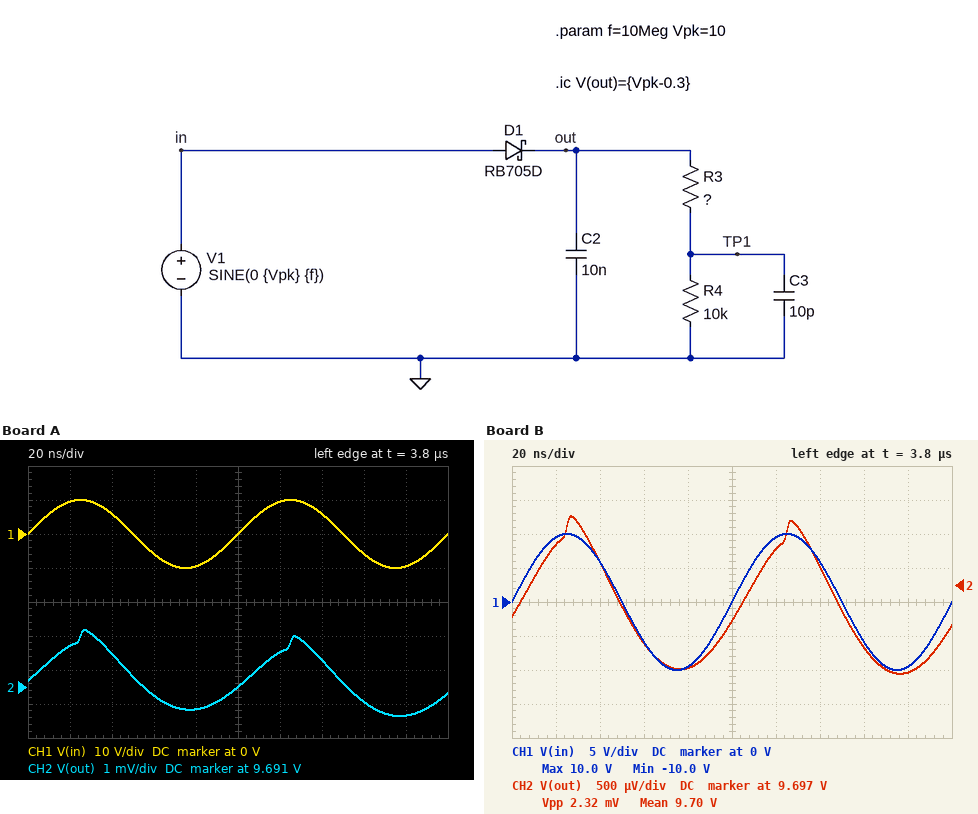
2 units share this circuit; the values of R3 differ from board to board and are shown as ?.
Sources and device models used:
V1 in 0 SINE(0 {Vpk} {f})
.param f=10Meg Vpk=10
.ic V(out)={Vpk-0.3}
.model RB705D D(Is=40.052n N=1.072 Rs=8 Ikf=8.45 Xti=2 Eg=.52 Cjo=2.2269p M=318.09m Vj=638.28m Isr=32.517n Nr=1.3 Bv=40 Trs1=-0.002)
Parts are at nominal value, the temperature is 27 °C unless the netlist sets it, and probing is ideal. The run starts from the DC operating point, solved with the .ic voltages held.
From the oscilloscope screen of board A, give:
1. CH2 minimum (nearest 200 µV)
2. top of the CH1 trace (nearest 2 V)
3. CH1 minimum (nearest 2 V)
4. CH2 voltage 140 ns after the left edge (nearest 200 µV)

9.6902 V
10 V
-10 V
9.6918 V
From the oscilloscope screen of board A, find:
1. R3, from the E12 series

150 kΩ
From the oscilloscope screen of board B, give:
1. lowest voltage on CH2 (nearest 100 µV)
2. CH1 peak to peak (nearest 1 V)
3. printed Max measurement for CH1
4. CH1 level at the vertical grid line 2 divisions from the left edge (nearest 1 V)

9.6962 V
20 V
10.0 V
6 V
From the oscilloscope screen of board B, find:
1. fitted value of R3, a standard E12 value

220 kΩ
